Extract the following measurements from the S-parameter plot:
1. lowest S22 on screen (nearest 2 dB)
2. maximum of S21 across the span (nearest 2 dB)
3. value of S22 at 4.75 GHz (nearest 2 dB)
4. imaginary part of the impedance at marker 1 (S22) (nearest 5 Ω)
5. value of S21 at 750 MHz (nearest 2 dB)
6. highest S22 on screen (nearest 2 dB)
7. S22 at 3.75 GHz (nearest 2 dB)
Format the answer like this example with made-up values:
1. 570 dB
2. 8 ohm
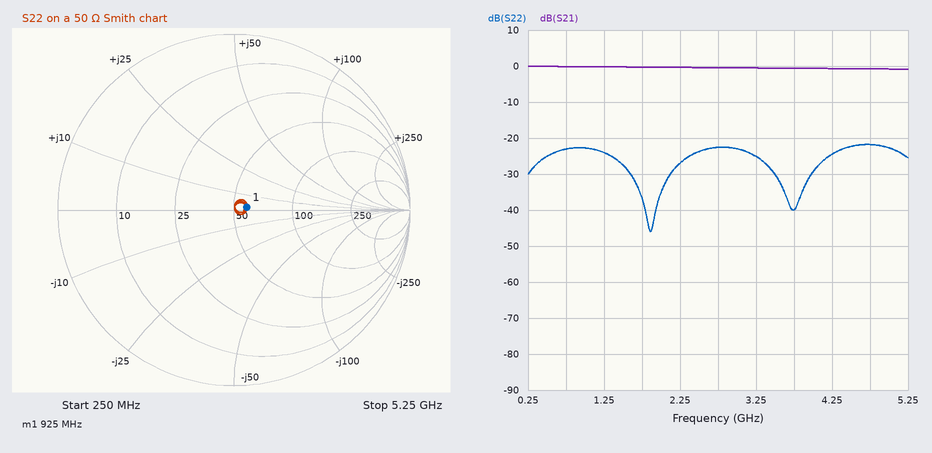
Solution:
1. -46 dB
2. 0 dB
3. -22 dB
4. 0 Ω
5. 0 dB
6. -22 dB
7. -40 dB
